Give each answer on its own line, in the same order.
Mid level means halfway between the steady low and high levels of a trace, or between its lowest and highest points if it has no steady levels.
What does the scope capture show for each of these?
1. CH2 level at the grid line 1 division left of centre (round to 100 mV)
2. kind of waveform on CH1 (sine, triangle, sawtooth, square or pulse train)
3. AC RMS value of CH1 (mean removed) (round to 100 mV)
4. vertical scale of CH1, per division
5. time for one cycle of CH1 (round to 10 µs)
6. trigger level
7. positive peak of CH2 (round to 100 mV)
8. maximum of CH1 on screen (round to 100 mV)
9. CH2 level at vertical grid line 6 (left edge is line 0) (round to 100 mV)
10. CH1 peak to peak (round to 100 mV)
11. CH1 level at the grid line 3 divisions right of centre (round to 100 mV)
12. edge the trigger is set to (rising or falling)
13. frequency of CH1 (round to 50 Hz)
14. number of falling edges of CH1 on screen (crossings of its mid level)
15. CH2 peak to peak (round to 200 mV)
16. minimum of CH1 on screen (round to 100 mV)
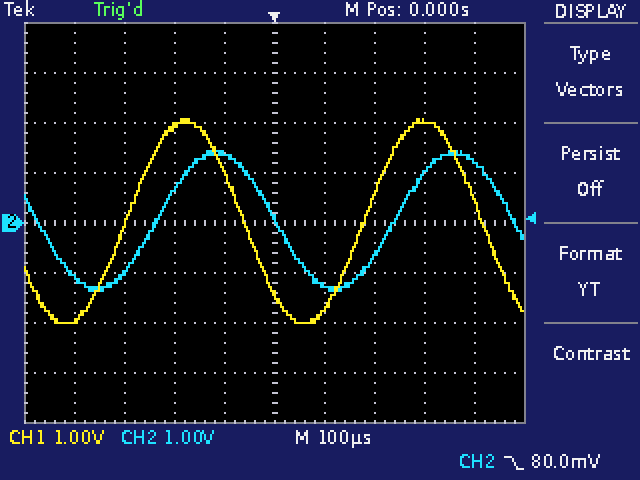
1.4 V
sine
1.4 V
1 V
480 µs
80.0 mV
1.4 V
2.1 V
-1.2 V
4.1 V
2.0 V
falling
2.10 kHz
2
2.8 V
-2.0 V
